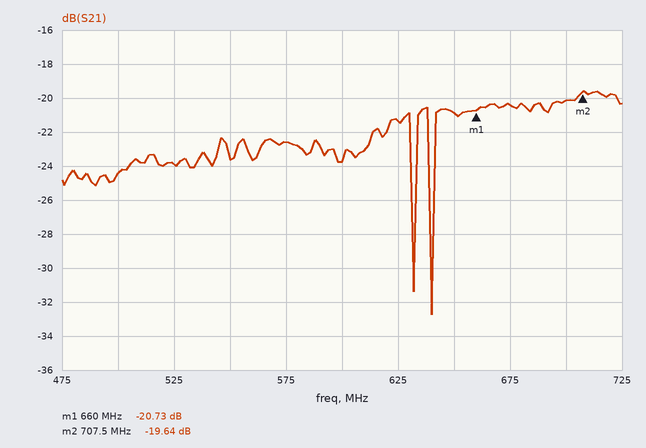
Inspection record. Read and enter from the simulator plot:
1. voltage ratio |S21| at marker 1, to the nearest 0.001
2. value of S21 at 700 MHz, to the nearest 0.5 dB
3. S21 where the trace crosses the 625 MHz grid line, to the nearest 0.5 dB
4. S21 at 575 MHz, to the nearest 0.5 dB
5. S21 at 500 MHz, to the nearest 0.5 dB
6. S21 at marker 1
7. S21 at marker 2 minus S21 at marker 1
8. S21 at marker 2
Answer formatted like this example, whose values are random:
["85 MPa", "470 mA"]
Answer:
["0.092", "-20.0 dB", "-21.5 dB", "-22.5 dB", "-24.5 dB", "-20.73 dB", "1.09 dB", "-19.64 dB"]
